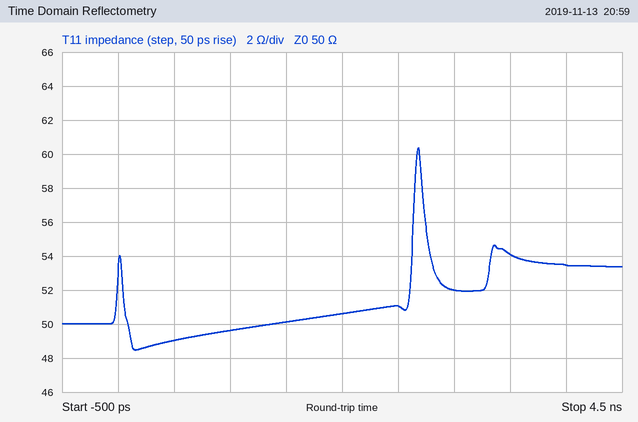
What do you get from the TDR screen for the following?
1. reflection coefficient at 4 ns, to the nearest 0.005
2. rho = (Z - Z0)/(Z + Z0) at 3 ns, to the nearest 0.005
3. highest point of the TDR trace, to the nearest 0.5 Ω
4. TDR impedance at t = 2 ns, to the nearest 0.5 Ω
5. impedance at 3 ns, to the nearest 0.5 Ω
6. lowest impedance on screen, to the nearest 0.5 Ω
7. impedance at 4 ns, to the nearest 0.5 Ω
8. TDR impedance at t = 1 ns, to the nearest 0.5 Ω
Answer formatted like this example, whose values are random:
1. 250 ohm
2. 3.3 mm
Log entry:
1. +0.035
2. +0.020
3. 60.5 Ω
4. 50.5 Ω
5. 52.0 Ω
6. 48.5 Ω
7. 53.5 Ω
8. 49.5 Ω
